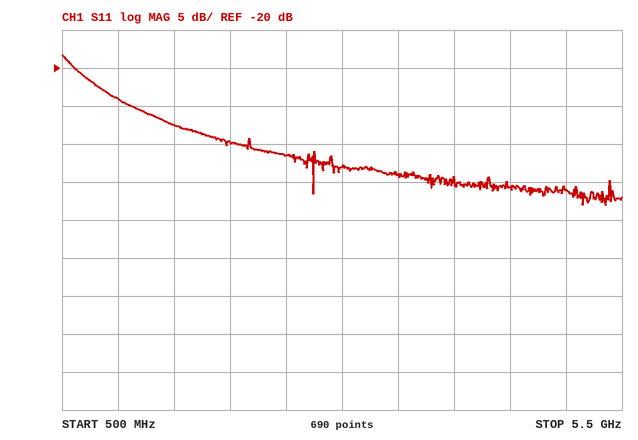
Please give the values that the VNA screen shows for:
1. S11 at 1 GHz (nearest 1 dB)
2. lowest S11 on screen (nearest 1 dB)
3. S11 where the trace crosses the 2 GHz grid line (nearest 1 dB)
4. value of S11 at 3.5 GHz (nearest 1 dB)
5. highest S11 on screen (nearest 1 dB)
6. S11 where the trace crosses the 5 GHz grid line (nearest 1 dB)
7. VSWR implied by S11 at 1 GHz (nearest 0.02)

-24 dB
-38 dB
-30 dB
-34 dB
-18 dB
-36 dB
1.14
